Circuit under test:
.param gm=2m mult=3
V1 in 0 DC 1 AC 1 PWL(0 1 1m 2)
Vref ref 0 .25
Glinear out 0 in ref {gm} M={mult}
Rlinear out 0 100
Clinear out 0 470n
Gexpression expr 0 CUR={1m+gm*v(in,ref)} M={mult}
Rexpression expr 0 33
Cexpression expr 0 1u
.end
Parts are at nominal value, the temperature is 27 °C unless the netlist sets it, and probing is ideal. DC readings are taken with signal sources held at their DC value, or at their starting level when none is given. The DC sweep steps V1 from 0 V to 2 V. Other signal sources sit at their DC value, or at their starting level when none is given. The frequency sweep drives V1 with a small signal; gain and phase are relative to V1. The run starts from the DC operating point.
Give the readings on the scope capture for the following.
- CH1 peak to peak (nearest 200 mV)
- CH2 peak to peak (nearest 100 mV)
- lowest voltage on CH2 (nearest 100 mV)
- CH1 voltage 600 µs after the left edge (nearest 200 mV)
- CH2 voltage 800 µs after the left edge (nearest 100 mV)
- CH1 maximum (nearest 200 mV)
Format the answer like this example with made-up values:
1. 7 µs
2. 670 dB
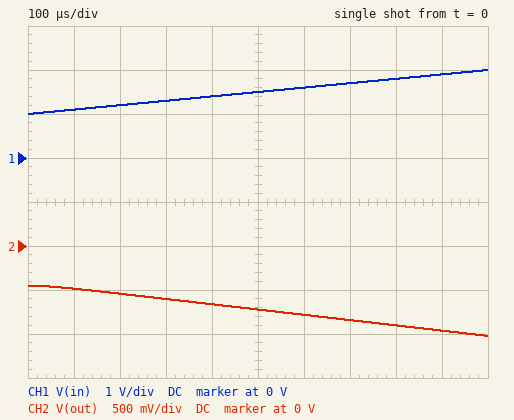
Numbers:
1. 1.0 V
2. 600 mV
3. -1.0 V
4. 1.6 V
5. -900 mV
6. 2.0 V
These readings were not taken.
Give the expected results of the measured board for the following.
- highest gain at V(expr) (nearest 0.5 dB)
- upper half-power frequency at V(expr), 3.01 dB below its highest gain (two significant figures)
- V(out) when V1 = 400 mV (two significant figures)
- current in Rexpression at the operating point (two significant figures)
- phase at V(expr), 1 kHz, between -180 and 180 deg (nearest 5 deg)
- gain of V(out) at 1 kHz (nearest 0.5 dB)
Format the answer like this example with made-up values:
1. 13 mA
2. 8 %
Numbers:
1. -14.0 dB
2. 4.8 kHz
3. -90 mV
4. 7.5 mA
5. 170 deg
6. -5.0 dB
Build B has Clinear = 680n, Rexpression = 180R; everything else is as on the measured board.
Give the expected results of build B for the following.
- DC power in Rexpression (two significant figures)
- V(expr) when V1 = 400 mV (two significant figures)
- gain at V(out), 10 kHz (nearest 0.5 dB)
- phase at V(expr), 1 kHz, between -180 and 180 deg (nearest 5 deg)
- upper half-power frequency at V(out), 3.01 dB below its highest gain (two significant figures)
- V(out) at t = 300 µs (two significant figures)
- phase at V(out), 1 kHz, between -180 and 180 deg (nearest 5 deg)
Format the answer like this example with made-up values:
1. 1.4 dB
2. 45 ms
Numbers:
1. 10 mW
2. -700 mV
3. -17.5 dB
4. 130 deg
5. 2.3 kHz
6. -590 mV
7. 155 deg
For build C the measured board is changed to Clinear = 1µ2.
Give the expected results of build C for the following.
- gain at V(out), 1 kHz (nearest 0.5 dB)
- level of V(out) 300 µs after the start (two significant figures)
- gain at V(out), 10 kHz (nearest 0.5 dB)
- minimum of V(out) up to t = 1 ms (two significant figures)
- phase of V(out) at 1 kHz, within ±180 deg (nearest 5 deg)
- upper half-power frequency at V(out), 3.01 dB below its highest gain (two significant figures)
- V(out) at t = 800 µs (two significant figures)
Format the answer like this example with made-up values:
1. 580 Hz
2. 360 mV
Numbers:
1. -6.5 dB
2. -560 mV
3. -22.0 dB
4. -980 mV
5. 145 deg
6. 1.3 kHz
7. -860 mV
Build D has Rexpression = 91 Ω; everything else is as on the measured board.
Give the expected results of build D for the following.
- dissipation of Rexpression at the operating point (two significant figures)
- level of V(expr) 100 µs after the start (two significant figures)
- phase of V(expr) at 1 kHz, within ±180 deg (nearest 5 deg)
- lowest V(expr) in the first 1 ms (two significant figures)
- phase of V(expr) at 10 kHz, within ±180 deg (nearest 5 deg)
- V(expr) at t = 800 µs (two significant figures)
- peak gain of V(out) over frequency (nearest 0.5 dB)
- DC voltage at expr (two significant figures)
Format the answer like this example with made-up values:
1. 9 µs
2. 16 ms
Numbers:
1. 5.1 mW
2. -700 mV
3. 150 deg
4. -1.2 V
5. 100 deg
6. -1.1 V
7. -4.5 dB
8. -680 mV
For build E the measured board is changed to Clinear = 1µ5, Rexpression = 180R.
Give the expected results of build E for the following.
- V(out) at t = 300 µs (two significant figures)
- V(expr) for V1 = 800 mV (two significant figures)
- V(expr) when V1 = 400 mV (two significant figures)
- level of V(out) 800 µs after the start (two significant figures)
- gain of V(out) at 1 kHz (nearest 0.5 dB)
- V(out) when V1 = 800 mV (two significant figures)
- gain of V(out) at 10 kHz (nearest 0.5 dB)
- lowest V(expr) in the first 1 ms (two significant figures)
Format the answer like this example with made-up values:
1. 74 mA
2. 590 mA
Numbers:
1. -550 mV
2. -1.1 V
3. -700 mV
4. -840 mV
5. -7.0 dB
6. -330 mV
7. -24.0 dB
8. -2.2 V
